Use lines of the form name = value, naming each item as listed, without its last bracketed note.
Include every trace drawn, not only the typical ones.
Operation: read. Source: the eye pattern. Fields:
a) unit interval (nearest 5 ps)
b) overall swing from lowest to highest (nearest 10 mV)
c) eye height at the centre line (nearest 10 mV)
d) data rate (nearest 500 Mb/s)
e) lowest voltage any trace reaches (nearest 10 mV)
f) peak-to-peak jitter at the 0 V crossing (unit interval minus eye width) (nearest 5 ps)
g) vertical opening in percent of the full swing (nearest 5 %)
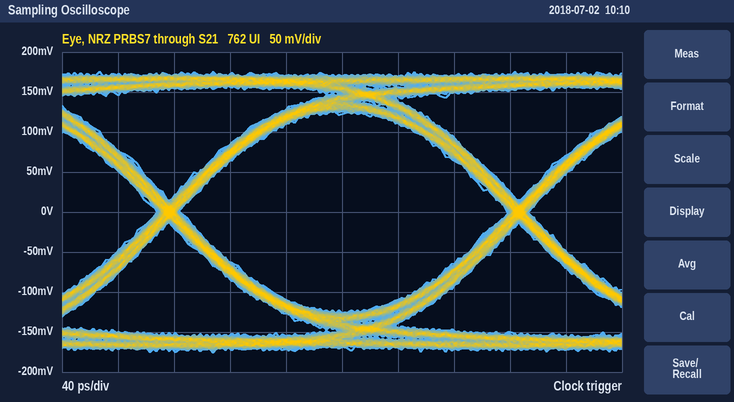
unit interval = 250 ps
overall swing from lowest to highest = 350 mV
eye height at the centre line = 250 mV
data rate = 4.0 Gb/s
lowest voltage any trace reaches = -180 mV
peak-to-peak jitter at the 0 V crossing (unit interval minus eye width) = 15 ps
vertical opening in percent of the full swing = 70 %
